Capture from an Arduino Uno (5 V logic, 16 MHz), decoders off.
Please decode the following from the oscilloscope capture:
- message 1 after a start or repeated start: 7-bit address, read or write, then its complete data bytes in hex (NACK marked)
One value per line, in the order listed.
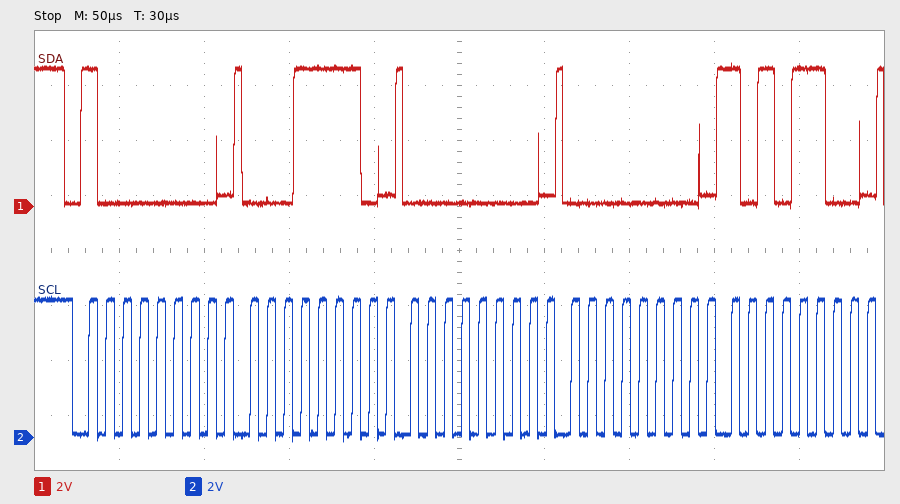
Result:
0x40 write: 1E 00 00 AC
